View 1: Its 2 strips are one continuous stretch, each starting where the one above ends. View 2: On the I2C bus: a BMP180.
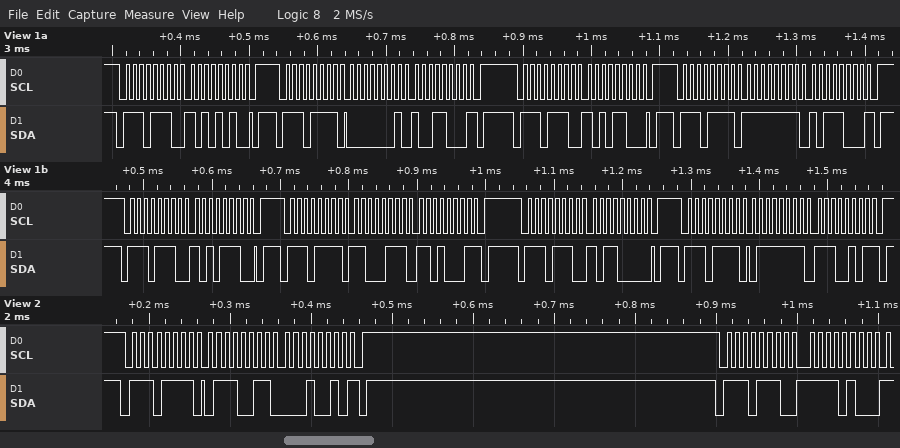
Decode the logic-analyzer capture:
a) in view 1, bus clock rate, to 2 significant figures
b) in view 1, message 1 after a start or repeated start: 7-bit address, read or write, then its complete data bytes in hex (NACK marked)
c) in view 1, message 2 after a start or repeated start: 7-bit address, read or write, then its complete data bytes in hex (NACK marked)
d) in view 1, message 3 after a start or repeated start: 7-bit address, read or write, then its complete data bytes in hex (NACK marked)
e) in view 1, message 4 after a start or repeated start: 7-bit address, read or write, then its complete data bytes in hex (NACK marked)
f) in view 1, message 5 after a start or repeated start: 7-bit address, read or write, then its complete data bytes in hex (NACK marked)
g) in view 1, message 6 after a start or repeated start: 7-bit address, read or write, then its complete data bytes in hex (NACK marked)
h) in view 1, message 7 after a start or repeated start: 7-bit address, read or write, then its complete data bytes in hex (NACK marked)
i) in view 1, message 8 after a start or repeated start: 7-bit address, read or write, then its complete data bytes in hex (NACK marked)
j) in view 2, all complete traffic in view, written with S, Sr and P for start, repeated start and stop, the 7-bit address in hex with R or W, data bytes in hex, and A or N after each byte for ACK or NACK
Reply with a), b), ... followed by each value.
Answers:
a) 100 kHz
b) 0x77 write: AA
c) 0x77 read: 01 98 NACK
d) 0x77 write: AC
e) 0x77 read: FF B8 NACK
f) 0x77 write: AE
g) 0x77 read: C7 D1 NACK
h) 0x77 write: B0
i) 0x77 read: 7F E5 NACK
j) S 77R A 73 A 12 N P S 77W A F4 A
